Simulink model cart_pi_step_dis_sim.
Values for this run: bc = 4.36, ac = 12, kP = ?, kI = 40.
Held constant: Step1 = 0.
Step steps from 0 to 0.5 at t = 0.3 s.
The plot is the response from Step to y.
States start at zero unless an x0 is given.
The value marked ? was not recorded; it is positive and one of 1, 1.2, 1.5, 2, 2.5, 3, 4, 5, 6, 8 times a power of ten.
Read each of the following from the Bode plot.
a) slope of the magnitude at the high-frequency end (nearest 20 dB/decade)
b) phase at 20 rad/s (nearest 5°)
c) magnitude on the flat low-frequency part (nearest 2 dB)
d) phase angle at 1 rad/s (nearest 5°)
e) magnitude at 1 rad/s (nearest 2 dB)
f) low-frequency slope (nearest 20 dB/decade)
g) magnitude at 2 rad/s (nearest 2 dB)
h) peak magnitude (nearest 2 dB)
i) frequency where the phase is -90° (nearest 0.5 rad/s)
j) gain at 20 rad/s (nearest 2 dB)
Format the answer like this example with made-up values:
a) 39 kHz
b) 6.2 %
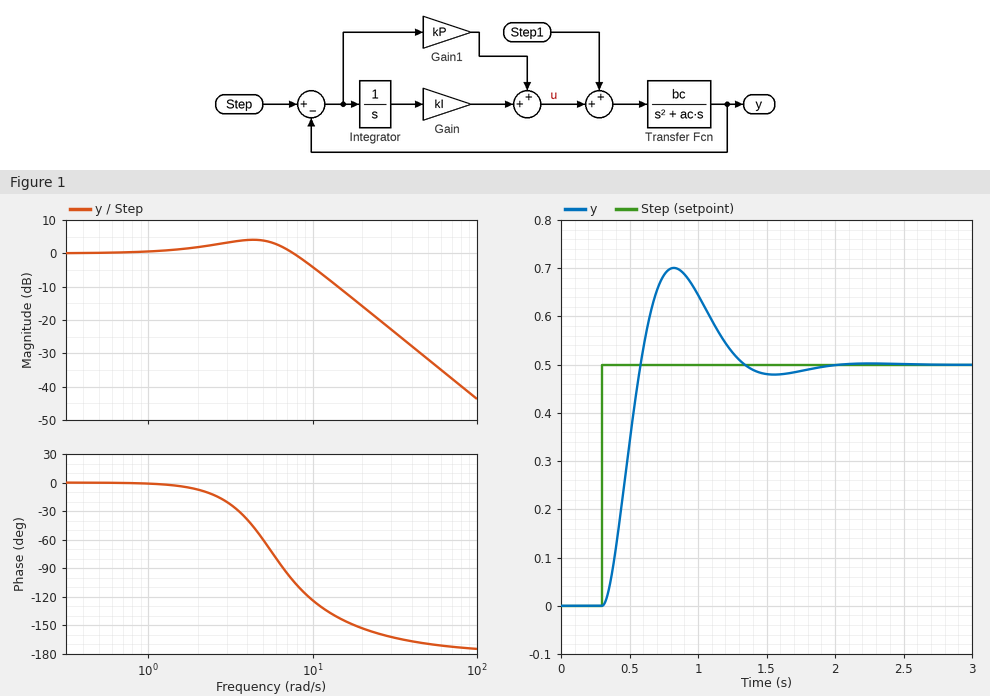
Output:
a) -40 dB/decade
b) -155°
c) 0 dB
d) 0°
e) 0 dB
f) 0 dB/decade
g) 2 dB
h) 4 dB
i) 6.5 rad/s
j) -16 dB
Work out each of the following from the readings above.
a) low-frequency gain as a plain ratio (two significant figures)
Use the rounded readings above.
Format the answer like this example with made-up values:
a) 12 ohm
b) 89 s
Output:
a) 1.0
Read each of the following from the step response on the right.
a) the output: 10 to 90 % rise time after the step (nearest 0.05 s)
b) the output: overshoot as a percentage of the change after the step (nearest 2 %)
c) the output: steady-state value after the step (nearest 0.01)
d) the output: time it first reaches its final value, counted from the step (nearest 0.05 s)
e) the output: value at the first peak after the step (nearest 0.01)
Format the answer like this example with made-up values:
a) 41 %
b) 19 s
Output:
a) 0.20 s
b) 40 %
c) 0.50
d) 0.30 s
e) 0.70
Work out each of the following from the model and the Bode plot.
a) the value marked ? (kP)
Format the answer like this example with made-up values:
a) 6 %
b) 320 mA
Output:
a) 15
